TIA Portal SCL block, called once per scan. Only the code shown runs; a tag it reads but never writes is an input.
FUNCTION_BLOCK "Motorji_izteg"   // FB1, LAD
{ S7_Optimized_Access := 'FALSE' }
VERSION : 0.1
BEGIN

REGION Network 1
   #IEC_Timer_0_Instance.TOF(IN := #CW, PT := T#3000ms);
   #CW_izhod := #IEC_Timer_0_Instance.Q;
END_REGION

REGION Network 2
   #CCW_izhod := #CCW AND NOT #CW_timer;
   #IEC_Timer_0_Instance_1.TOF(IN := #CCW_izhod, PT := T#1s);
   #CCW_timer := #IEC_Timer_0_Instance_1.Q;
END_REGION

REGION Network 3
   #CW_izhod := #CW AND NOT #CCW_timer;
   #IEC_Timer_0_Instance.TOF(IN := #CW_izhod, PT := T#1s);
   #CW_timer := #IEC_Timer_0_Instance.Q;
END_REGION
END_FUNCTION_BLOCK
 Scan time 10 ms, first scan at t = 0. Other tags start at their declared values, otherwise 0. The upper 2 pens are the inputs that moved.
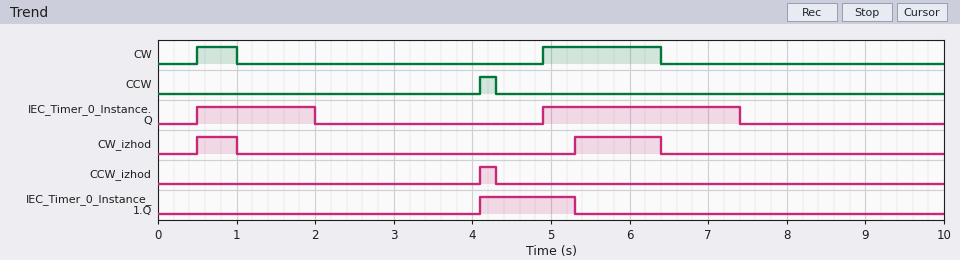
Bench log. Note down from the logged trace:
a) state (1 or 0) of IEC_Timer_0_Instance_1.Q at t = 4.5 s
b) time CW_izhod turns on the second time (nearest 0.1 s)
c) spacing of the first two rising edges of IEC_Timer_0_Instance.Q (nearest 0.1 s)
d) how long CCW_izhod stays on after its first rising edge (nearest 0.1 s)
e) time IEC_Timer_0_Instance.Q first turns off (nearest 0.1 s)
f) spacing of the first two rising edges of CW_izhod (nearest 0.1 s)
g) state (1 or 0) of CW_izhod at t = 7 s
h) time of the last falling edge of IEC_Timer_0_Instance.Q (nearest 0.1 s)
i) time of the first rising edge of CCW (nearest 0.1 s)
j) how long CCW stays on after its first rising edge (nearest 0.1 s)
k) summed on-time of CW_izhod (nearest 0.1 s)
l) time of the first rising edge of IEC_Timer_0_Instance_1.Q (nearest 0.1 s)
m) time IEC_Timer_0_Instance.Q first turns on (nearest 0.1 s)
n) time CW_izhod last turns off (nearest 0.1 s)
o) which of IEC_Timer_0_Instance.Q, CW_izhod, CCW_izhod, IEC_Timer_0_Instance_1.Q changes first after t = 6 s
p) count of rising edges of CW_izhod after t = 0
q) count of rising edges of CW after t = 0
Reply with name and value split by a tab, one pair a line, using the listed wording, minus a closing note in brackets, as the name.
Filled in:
state (1 or 0) of IEC_Timer_0_Instance_1.Q at t = 4.5 s	1
time CW_izhod turns on the second time	5.3 s
spacing of the first two rising edges of IEC_Timer_0_Instance.Q	4.4 s
how long CCW_izhod stays on after its first rising edge	0.2 s
time IEC_Timer_0_Instance.Q first turns off	2.0 s
spacing of the first two rising edges of CW_izhod	4.8 s
state (1 or 0) of CW_izhod at t = 7 s	0
time of the last falling edge of IEC_Timer_0_Instance.Q	7.4 s
time of the first rising edge of CCW	4.1 s
how long CCW stays on after its first rising edge	0.2 s
summed on-time of CW_izhod	1.6 s
time of the first rising edge of IEC_Timer_0_Instance_1.Q	4.1 s
time IEC_Timer_0_Instance.Q first turns on	0.5 s
time CW_izhod last turns off	6.4 s
which of IEC_Timer_0_Instance.Q, CW_izhod, CCW_izhod, IEC_Timer_0_Instance_1.Q changes first after t = 6 s	CW_izhod
count of rising edges of CW_izhod after t = 0	2
count of rising edges of CW after t = 0	2
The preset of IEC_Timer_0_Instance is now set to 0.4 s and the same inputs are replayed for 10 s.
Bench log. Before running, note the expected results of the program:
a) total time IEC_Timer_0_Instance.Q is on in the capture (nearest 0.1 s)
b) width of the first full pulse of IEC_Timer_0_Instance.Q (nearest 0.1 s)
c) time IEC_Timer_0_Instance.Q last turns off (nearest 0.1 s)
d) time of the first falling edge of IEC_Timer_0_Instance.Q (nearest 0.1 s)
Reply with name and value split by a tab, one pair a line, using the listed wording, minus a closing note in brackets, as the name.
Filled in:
total time IEC_Timer_0_Instance.Q is on in the capture	2.8 s
width of the first full pulse of IEC_Timer_0_Instance.Q	0.9 s
time IEC_Timer_0_Instance.Q last turns off	6.8 s
time of the first falling edge of IEC_Timer_0_Instance.Q	1.4 s
